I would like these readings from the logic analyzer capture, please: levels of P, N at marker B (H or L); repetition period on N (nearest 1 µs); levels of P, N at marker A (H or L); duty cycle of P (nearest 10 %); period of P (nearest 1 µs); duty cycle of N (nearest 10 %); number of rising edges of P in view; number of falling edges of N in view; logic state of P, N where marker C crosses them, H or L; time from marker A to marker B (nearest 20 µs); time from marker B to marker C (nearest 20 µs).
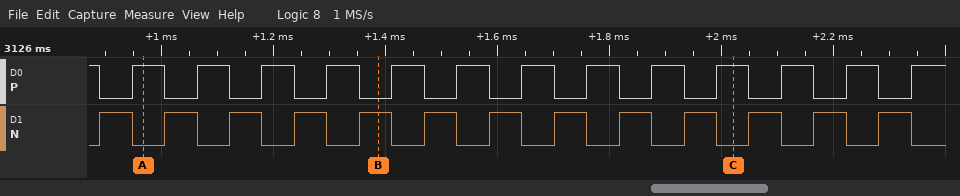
P=L, N=H
116 µs
P=H, N=L
50 %
116 µs
50 %
13
13
P=H, N=L
420 µs
640 µs
